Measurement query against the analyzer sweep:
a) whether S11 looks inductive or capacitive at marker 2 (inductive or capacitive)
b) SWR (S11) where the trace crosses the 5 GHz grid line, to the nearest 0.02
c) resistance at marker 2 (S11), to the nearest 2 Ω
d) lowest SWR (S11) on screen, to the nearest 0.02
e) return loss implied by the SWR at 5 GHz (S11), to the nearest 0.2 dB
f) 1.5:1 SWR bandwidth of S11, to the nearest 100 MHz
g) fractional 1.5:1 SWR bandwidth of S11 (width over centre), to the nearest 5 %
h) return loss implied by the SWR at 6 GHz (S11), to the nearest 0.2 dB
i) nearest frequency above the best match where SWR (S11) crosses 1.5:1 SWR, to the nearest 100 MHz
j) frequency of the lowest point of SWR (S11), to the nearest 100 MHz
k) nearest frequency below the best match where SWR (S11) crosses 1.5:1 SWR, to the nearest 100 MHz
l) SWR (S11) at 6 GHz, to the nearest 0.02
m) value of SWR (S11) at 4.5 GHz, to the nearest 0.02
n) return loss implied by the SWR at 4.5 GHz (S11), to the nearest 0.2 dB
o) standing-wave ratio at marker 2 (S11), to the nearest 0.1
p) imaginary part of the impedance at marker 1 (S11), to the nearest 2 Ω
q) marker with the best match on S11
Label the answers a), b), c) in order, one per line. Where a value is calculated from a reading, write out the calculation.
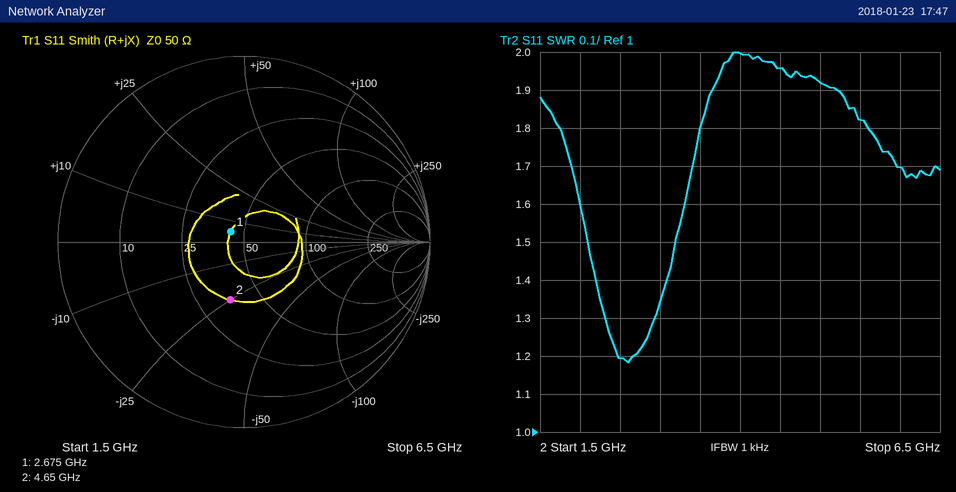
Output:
a) capacitive
b) 1.92
c) 36 Ω
d) 1.18
e) −20 log10((1.92 − 1)/(1.92 + 1)) ≈ 10.0 dB
f) 3.2 GHz − 2.1 GHz = 1.1 GHz
g) 1.1 GHz / 2.65 GHz ≈ 41.5 %, so 40 % to the nearest 5 %
h) −20 log10((1.7 − 1)/(1.7 + 1)) ≈ 11.7 dB, so 11.8 dB to the nearest 0.2 dB
i) 3.2 GHz
j) 2.6 GHz
k) 2.1 GHz
l) 1.70
m) 1.96
n) −20 log10((1.96 − 1)/(1.96 + 1)) ≈ 9.8 dB
o) 1.9
p) +4 Ω
q) marker 1
